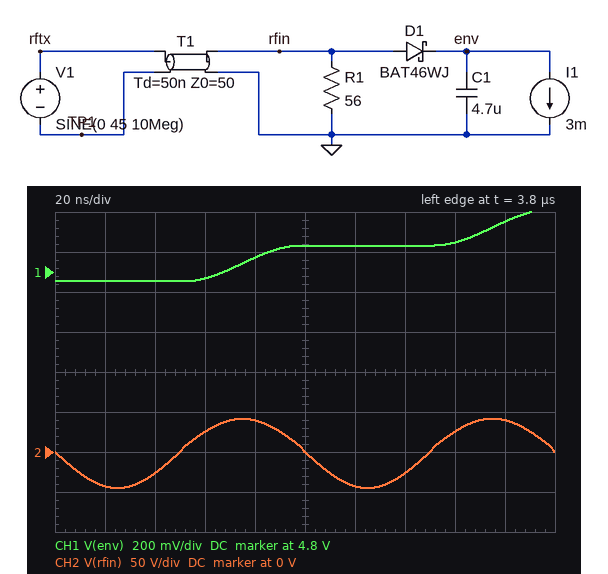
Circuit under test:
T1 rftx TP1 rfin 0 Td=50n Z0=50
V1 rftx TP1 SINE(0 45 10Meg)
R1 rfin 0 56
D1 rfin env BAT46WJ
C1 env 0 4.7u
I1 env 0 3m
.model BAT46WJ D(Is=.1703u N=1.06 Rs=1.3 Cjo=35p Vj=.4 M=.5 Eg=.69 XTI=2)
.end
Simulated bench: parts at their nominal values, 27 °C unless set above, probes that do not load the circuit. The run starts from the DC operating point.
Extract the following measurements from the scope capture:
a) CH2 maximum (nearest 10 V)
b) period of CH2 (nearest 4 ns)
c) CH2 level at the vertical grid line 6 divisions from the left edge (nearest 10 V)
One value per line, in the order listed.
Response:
40 V
100 ns
-40 V
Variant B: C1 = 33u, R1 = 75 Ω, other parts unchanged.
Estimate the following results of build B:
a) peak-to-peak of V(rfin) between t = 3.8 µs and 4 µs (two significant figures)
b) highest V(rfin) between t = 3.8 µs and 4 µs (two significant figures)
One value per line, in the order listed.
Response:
85 V
40 V
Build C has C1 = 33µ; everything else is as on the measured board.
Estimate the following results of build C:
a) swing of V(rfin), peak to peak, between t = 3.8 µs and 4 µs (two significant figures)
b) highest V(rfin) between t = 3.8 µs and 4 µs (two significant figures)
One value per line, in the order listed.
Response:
85 V
40 V
